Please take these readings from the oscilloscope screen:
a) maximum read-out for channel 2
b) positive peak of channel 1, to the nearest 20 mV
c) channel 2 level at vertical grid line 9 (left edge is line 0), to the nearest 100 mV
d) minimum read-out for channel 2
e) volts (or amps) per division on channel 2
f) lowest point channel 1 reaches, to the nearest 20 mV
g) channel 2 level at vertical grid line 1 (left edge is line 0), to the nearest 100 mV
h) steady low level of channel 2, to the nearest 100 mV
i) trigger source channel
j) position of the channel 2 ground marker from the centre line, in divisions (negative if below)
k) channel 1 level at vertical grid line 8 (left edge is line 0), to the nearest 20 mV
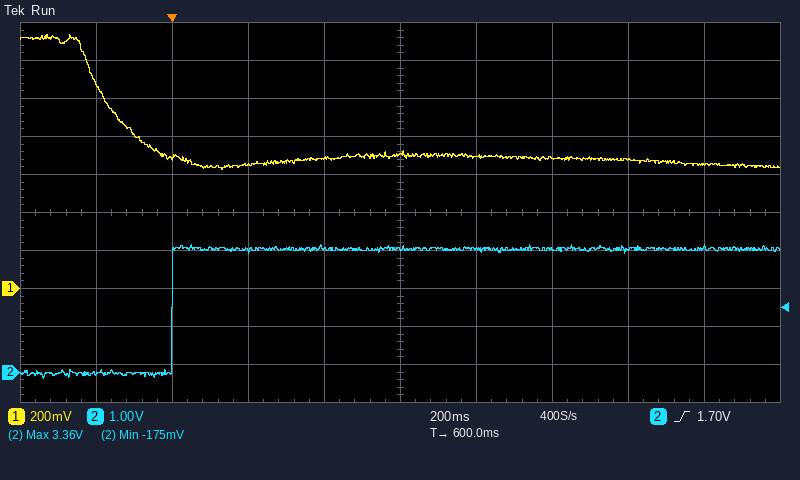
3.36 V
1.34 V
3.3 V
-175 mV
1 V
620 mV
0.0 V
0.0 V
channel 2
-4.2 div
680 mV
